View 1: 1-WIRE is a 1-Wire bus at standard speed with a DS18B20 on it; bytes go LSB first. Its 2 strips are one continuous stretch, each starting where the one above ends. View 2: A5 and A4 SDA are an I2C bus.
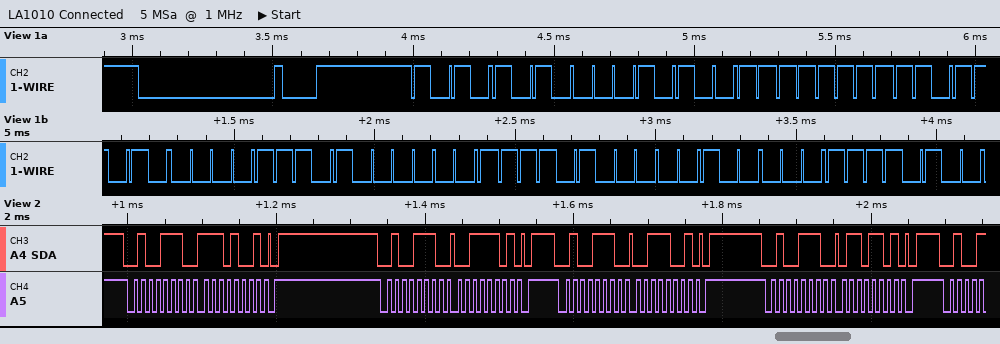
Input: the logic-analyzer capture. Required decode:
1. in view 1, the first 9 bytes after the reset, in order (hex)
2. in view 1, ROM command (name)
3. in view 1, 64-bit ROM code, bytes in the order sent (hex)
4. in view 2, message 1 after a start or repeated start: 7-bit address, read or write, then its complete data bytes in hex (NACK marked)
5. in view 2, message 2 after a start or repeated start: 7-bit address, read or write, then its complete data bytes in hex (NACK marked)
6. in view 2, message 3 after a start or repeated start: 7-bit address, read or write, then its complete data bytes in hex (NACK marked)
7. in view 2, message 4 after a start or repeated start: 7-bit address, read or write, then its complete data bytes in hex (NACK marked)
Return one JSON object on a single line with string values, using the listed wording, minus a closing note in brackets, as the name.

{"in view 1, the first 9 bytes after the reset, in order": "55 28 FF 5B 70 81 17 04 2F", "in view 1, ROM command": "Match ROM", "in view 1, 64-bit ROM code, bytes in the order sent": "28 FF 5B 70 81 17 04 2F", "in view 2, message 1 after a start or repeated start: 7-bit address, read or write, then its complete data bytes in hex": "0x27 write: E9", "in view 2, message 2 after a start or repeated start: 7-bit address, read or write, then its complete data bytes in hex": "0x27 write: 3D", "in view 2, message 3 after a start or repeated start: 7-bit address, read or write, then its complete data bytes in hex": "0x27 write: 39", "in view 2, message 4 after a start or repeated start: 7-bit address, read or write, then its complete data bytes in hex": "0x27 write: 6D"}
